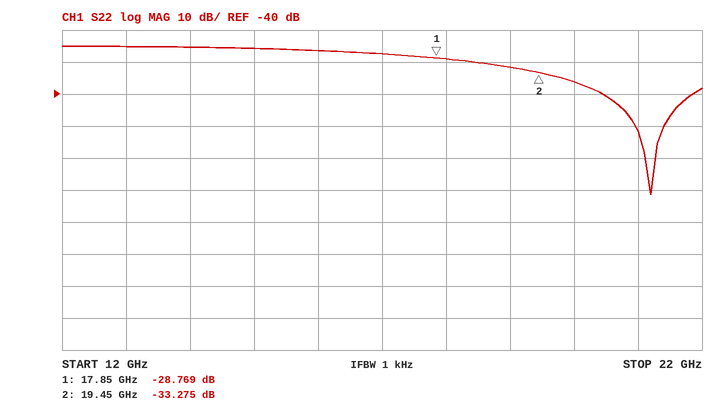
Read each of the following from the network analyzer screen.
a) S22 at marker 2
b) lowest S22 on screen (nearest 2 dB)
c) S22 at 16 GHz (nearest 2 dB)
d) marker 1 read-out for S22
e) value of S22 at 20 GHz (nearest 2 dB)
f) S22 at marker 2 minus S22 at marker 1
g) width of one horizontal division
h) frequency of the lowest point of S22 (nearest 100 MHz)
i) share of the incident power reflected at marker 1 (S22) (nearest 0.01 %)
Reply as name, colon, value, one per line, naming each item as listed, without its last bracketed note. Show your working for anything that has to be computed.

S22 at marker 2: -33.275 dB
lowest S22 on screen: -72 dB
S22 at 16 GHz: -26 dB
marker 1 read-out for S22: -28.769 dB
value of S22 at 20 GHz: -36 dB
S22 at marker 2 minus S22 at marker 1: -33.275 − (-28.769) = -4.506 dB
width of one horizontal division: 1 GHz
frequency of the lowest point of S22: 21.2 GHz
share of the incident power reflected at marker 1 (S22): 10^(-28.769/10) ≈ 0.13 %
